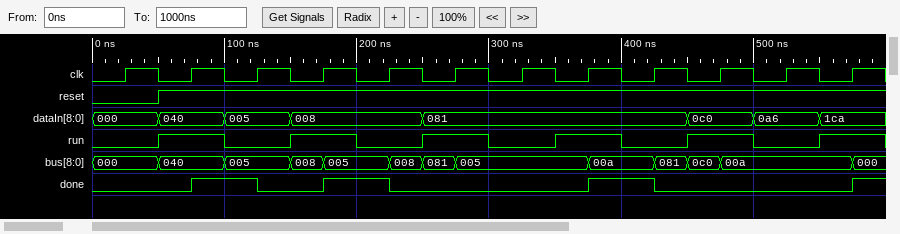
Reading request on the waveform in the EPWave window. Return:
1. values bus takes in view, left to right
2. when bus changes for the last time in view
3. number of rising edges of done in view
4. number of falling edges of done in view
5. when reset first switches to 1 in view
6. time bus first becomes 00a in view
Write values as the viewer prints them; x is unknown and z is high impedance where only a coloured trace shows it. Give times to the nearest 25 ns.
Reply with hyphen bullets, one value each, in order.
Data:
- 000, 040, 005, 008, 005, 008, 081, 005, 00a, 081, 0c0, 00a, 000
- 575 ns
- 4
- 3
- 50 ns
- 375 ns
